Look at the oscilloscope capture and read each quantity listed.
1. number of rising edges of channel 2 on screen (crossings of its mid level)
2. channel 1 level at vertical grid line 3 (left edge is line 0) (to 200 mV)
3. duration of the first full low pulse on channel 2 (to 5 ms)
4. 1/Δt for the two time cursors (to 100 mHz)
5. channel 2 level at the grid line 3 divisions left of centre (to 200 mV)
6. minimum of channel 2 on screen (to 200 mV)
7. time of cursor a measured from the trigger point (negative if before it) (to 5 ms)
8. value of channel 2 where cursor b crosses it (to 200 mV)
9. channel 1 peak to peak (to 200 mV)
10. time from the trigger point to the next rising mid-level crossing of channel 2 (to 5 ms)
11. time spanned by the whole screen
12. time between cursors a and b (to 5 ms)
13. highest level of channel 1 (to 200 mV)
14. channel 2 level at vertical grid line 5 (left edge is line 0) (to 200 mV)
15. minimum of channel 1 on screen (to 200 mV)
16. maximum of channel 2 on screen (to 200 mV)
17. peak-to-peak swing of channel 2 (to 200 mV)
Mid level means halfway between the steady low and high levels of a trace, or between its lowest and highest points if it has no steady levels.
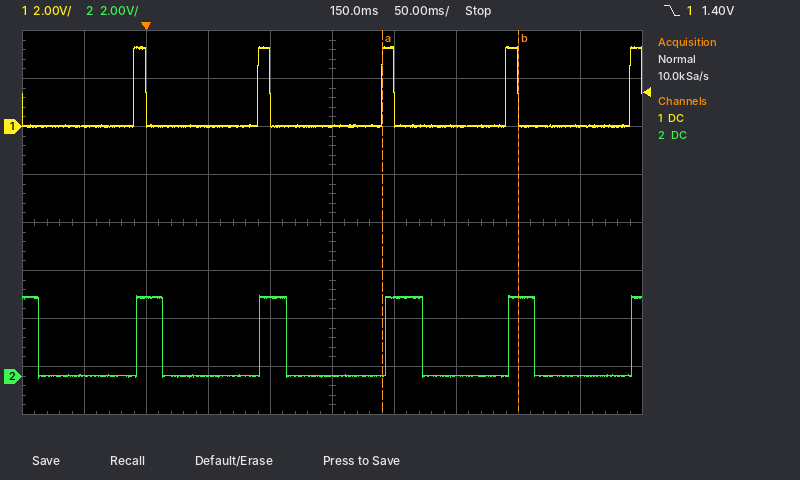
5
0.0 V
80 ms
9.1 Hz
3.2 V
0.0 V
+190 ms
3.2 V
3.4 V
90 ms
500 ms
110 ms
3.4 V
0.0 V
0.0 V
3.4 V
3.4 V
